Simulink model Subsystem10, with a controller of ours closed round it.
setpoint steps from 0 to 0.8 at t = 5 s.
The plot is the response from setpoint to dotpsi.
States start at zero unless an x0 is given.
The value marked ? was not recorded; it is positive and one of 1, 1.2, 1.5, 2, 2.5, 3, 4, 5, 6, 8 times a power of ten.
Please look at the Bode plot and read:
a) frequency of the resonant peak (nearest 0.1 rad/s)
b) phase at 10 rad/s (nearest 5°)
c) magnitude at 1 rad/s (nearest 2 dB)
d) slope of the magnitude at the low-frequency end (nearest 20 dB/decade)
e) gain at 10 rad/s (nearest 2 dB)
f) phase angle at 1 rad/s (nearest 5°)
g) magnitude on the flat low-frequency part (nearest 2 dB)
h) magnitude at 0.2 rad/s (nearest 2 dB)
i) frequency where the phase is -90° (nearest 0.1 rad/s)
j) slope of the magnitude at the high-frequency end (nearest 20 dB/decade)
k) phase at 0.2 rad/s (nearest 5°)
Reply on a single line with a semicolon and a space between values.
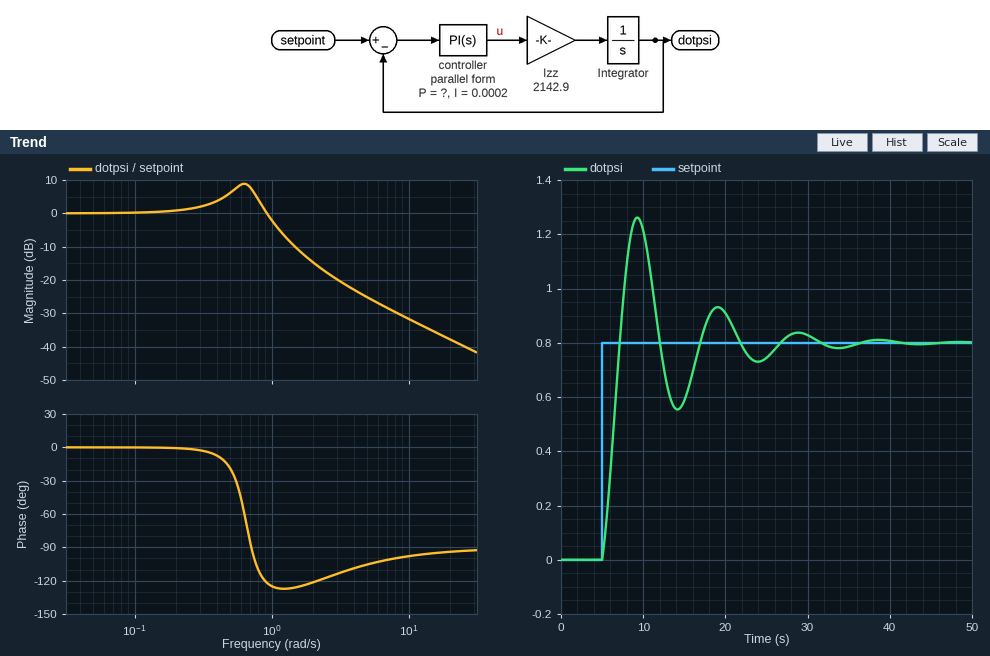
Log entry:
0.6 rad/s; -100°; -2 dB; 0 dB/decade; -32 dB; -125°; 0 dB; 0 dB; 0.7 rad/s; -20 dB/decade; 0°
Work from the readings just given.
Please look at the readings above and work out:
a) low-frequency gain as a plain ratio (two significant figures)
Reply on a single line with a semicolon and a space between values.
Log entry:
1.0
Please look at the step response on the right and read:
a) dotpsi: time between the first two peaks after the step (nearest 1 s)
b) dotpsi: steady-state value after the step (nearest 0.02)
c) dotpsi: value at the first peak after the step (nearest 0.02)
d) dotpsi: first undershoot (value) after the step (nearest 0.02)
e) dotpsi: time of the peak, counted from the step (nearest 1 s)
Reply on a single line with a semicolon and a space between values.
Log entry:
10 s; 0.80; 1.26; 0.56; 4 s
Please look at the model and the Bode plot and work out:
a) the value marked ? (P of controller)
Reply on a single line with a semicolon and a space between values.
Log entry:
0.00012
